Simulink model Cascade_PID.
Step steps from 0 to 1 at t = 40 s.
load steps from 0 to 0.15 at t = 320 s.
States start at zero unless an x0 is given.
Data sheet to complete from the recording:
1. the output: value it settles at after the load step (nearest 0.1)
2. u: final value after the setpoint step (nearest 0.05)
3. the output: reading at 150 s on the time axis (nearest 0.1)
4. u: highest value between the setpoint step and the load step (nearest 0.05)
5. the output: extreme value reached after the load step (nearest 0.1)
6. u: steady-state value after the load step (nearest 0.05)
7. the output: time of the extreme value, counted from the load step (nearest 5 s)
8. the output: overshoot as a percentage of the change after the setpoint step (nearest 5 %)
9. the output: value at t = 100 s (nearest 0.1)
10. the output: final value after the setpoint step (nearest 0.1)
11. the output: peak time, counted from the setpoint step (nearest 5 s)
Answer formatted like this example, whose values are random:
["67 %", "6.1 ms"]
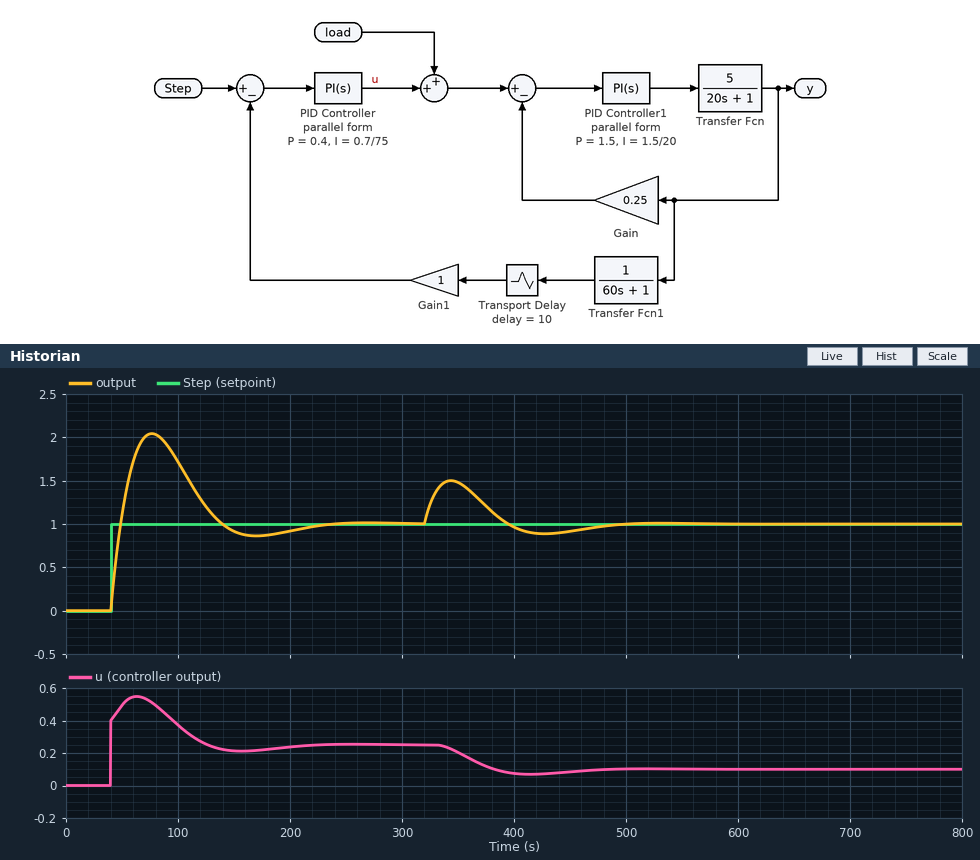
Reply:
["1.0", "0.25", "0.9", "0.55", "1.5", "0.10", "25 s", "105 %", "1.7", "1.0", "35 s"]
